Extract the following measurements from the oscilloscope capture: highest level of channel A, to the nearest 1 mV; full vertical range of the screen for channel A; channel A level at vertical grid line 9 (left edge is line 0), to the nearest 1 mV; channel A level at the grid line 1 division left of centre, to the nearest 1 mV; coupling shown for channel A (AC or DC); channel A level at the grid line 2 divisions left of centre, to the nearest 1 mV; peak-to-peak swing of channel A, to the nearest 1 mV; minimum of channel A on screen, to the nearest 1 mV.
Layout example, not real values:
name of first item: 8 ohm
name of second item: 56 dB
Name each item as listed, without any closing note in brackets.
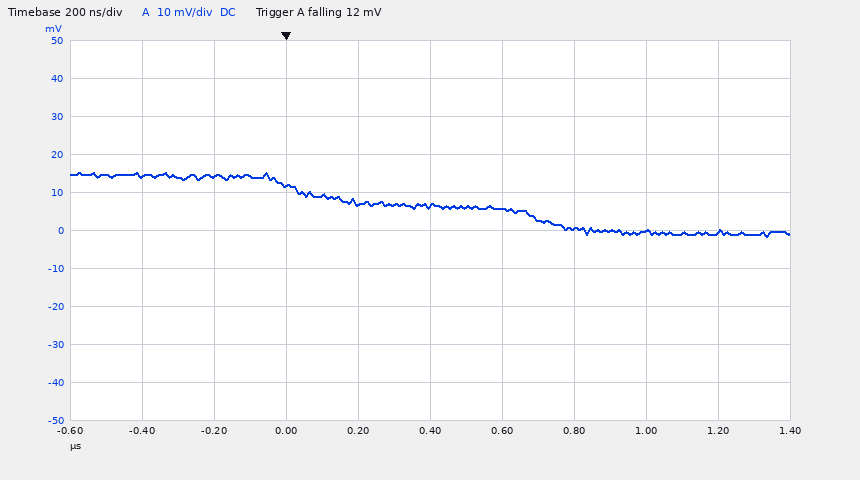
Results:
highest level of channel A, to the nearest 1 mV: 15 mV
full vertical range of the screen for channel A: 100 mV
channel A level at vertical grid line 9 (left edge is line 0), to the nearest 1 mV: 0 mV
channel A level at the grid line 1 division left of centre, to the nearest 1 mV: 7 mV
coupling shown for channel A: DC
channel A level at the grid line 2 divisions left of centre, to the nearest 1 mV: 12 mV
peak-to-peak swing of channel A, to the nearest 1 mV: 17 mV
minimum of channel A on screen, to the nearest 1 mV: -2 mV
